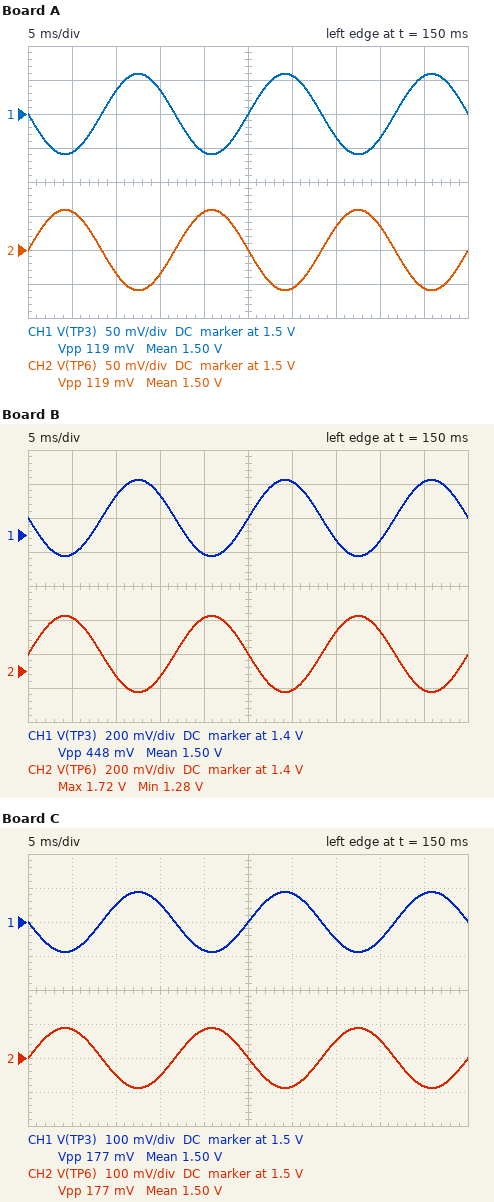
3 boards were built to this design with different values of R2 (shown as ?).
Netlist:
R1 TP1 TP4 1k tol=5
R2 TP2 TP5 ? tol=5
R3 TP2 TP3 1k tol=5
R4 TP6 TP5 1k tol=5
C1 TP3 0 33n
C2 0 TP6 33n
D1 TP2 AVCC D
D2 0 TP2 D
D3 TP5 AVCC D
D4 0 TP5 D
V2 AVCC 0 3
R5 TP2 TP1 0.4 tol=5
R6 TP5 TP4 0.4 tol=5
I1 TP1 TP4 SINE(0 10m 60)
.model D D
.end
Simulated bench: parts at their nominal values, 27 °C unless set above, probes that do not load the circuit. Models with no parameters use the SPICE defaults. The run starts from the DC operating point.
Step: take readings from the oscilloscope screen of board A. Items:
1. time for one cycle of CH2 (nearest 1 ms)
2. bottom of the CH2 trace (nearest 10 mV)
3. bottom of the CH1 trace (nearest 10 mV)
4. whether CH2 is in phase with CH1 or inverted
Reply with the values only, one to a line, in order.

17 ms
1.44 V
1.44 V
inverted
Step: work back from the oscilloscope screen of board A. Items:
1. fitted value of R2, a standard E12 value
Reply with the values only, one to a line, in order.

12 Ω
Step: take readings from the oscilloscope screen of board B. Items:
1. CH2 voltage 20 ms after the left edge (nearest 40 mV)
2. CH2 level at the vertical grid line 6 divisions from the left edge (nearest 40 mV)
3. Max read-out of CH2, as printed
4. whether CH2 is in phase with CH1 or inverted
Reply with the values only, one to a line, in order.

1.72 V
1.28 V
1.72 V
inverted
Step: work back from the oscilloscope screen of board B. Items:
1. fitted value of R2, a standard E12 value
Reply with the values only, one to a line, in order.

47 Ω
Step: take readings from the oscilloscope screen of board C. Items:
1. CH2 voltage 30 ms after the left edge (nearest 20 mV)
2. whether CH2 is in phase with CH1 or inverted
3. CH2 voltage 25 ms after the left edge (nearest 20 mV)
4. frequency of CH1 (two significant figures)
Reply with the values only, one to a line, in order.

1.42 V
inverted
1.50 V
60 Hz
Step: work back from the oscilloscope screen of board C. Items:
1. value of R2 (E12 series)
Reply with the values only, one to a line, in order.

18 Ω
